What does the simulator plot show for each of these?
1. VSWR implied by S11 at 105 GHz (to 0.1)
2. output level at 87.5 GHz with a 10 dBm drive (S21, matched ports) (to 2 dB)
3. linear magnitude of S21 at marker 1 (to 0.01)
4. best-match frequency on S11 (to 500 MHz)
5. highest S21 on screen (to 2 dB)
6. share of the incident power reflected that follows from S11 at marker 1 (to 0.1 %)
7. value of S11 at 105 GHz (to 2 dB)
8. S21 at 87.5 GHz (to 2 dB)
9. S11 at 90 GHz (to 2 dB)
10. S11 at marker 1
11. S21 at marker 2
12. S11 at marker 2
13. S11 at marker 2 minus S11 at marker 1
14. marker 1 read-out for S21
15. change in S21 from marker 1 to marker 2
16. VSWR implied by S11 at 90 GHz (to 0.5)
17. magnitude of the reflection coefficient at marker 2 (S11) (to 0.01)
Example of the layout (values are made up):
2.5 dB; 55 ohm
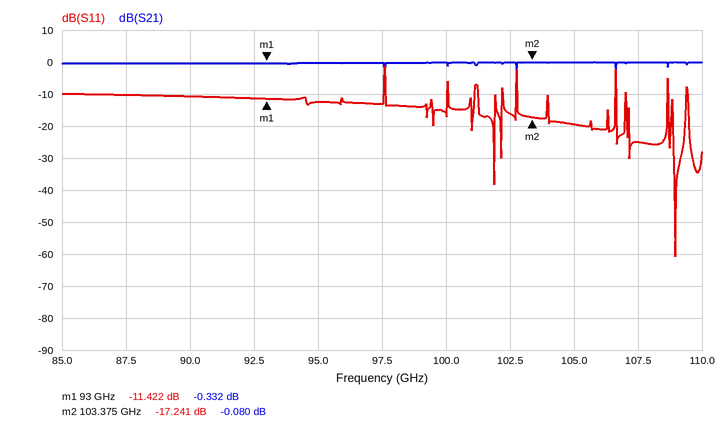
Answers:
1.2; 10 dBm; 0.96; 109.0 GHz; 0 dB; 7.2 %; -20 dB; 0 dB; -10 dB; -11.422 dB; -0.080 dB; -17.241 dB; -5.819 dB; -0.332 dB; 0.252 dB; 2.0; 0.14
